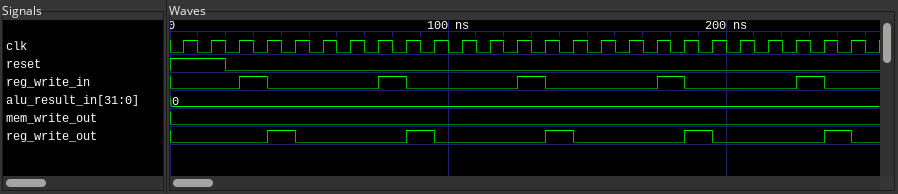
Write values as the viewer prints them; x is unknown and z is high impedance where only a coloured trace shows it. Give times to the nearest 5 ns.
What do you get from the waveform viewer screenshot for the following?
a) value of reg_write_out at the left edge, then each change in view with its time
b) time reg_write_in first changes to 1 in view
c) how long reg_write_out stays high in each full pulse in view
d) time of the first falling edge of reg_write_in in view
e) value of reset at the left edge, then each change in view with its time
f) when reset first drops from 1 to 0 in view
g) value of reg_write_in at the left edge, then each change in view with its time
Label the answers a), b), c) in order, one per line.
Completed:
a) 0, 1 at 35 ns, 0 at 45 ns, 1 at 85 ns, 0 at 95 ns, 1 at 135 ns, 0 at 145 ns, 1 at 185 ns, 0 at 195 ns, 1 at 235 ns, 0 at 245 ns
b) 25 ns
c) 10 ns, 10 ns, 10 ns, 10 ns, 10 ns
d) 35 ns
e) 1, 0 at 20 ns
f) 20 ns
g) 0, 1 at 25 ns, 0 at 35 ns, 1 at 75 ns, 0 at 85 ns, 1 at 125 ns, 0 at 135 ns, 1 at 175 ns, 0 at 185 ns, 1 at 225 ns, 0 at 235 ns
